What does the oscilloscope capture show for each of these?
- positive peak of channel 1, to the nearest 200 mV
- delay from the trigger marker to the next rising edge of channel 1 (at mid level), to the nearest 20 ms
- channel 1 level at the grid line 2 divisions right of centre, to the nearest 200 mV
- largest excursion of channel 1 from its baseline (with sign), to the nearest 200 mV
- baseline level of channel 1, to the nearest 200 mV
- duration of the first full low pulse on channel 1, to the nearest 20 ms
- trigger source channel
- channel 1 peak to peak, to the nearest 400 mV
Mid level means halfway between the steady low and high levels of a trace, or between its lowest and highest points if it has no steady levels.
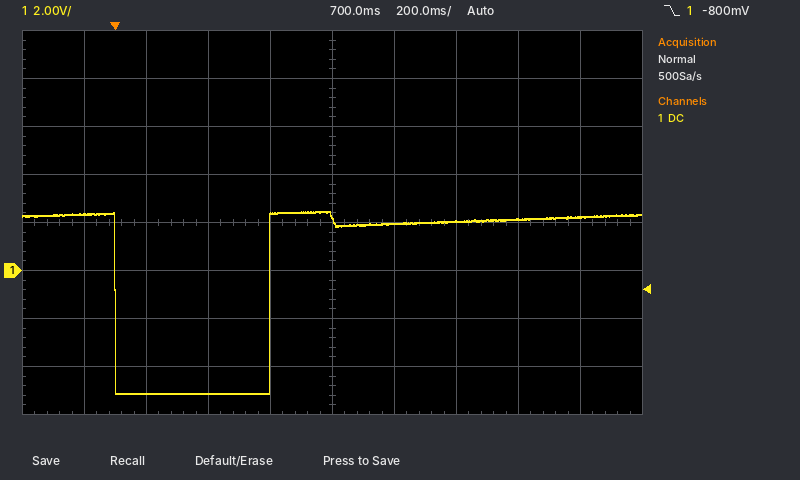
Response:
2.4 V
500 ms
2.0 V
-7.2 V
2.2 V
500 ms
channel 1
7.6 V
